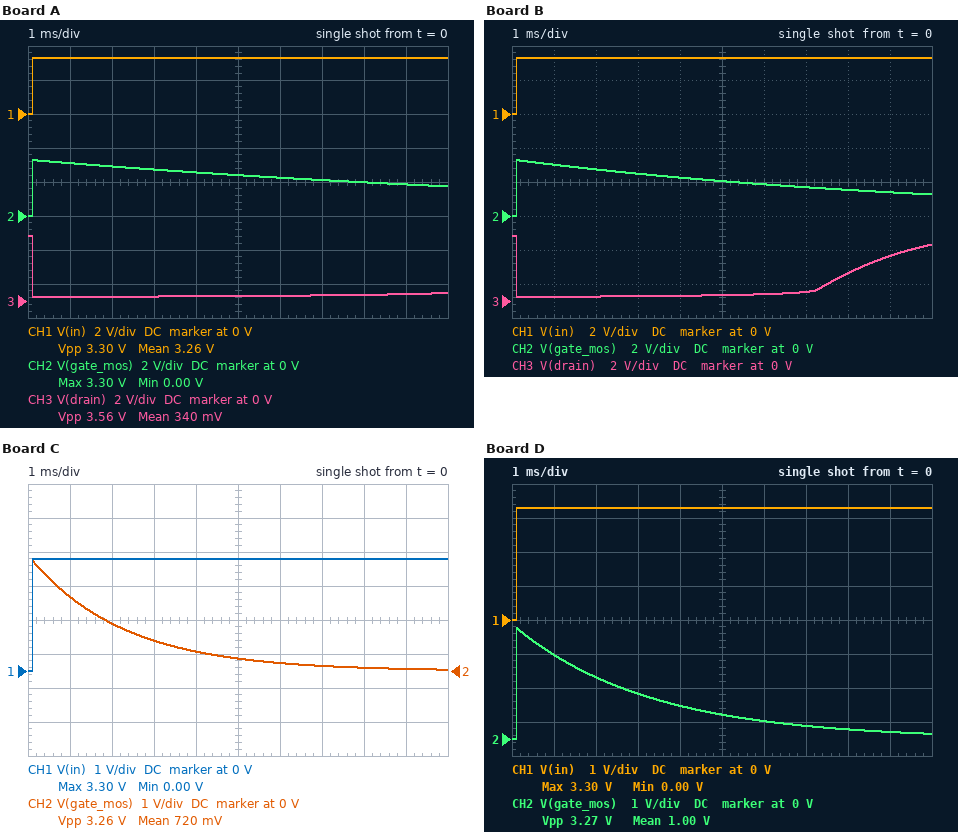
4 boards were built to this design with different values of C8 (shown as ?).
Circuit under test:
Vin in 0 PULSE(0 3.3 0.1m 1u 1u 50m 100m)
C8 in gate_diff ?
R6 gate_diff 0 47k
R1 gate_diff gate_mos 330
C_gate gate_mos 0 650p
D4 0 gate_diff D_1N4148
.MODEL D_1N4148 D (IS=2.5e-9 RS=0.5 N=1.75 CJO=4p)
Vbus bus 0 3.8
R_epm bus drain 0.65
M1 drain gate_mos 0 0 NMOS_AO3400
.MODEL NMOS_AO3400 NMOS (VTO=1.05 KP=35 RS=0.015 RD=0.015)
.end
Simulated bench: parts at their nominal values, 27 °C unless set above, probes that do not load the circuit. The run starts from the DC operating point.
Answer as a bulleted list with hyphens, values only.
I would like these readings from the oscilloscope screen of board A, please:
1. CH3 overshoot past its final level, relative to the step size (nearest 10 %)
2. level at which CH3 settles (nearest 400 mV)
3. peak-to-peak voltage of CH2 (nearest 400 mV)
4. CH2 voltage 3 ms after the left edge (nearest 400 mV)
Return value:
- 10 %
- 400 mV
- 3.2 V
- 2.8 V
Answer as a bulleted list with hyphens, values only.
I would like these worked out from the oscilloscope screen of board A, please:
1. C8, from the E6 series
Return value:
- 330 nF
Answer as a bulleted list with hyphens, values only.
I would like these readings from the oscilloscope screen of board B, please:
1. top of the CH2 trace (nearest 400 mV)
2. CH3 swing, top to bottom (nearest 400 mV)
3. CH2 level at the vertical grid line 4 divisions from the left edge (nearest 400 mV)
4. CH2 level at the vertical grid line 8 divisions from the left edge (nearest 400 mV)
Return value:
- 3.2 V
- 3.6 V
- 2.4 V
- 1.6 V
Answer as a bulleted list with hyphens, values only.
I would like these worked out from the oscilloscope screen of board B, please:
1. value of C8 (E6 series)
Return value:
- 220 nF
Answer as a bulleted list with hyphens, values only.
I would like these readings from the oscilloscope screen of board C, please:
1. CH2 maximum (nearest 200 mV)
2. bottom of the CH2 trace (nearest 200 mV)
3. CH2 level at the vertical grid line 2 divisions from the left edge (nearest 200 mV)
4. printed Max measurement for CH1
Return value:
- 3.2 V
- 0 V
- 1.4 V
- 3.30 V
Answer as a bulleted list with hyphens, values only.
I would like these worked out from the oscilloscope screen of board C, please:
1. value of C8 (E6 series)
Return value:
- 47 nF
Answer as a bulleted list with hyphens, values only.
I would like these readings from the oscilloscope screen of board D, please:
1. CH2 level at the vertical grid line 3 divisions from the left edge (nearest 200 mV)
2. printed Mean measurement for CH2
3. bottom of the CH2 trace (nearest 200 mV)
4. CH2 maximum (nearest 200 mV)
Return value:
- 1.4 V
- 1.00 V
- 0 V
- 3.2 V
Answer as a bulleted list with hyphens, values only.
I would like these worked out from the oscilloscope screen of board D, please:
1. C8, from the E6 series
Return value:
- 68 nF
